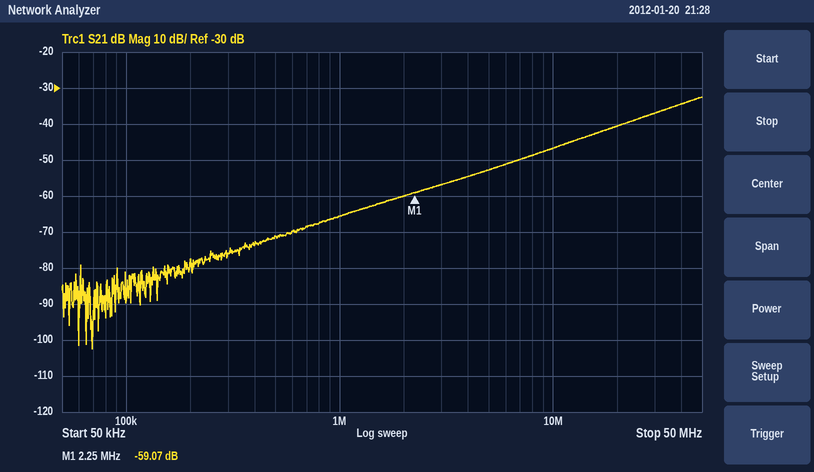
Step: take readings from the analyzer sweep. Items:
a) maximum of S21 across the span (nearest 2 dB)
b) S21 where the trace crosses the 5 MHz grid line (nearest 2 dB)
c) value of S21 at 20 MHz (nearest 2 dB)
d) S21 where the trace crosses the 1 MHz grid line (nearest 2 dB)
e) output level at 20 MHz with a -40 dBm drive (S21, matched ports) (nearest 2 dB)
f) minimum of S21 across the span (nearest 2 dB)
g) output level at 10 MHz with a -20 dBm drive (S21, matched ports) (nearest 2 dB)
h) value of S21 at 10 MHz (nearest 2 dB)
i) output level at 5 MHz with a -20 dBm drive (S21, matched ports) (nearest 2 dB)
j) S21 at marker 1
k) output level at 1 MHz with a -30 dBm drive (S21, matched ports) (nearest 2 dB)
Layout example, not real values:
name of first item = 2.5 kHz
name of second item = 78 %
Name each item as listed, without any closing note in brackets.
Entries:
maximum of S21 across the span = -32 dB
S21 where the trace crosses the 5 MHz grid line = -52 dB
value of S21 at 20 MHz = -40 dB
S21 where the trace crosses the 1 MHz grid line = -66 dB
output level at 20 MHz with a -40 dBm drive (S21, matched ports) = -80 dBm
minimum of S21 across the span = -102 dB
output level at 10 MHz with a -20 dBm drive (S21, matched ports) = -66 dBm
value of S21 at 10 MHz = -46 dB
output level at 5 MHz with a -20 dBm drive (S21, matched ports) = -72 dBm
S21 at marker 1 = -59.07 dB
output level at 1 MHz with a -30 dBm drive (S21, matched ports) = -96 dBm
